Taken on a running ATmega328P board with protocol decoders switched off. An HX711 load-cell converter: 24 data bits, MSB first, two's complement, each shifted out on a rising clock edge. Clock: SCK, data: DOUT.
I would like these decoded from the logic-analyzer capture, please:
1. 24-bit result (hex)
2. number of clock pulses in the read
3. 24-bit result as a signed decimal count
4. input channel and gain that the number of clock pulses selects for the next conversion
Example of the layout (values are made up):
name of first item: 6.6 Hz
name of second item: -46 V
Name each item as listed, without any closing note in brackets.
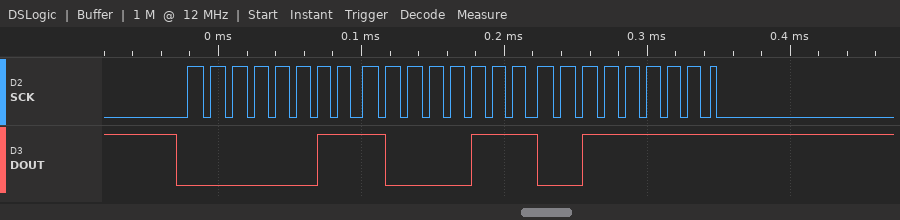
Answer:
24-bit result: 0x03873F
number of clock pulses in the read: 25
24-bit result as a signed decimal count: 231231
input channel and gain that the number of clock pulses selects for the next conversion: channel A, gain 128
